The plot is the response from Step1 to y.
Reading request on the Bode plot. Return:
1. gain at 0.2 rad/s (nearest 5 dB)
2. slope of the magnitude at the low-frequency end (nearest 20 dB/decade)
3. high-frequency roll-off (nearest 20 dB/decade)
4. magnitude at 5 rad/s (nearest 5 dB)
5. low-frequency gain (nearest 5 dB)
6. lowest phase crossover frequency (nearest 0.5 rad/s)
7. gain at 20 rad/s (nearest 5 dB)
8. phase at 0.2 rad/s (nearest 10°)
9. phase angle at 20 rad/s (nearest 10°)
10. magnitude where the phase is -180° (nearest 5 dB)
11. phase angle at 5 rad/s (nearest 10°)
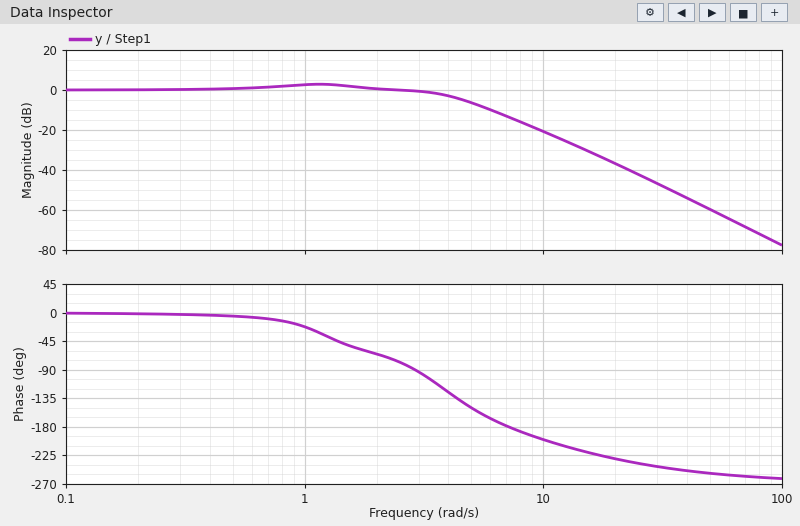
0 dB
0 dB/decade
-60 dB/decade
-5 dB
0 dB
7.0 rad/s
-35 dB
0°
-230°
-15 dB
-150°
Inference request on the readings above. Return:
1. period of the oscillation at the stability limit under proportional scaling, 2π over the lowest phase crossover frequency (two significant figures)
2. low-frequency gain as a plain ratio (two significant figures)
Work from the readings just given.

0.90 s
1.0
